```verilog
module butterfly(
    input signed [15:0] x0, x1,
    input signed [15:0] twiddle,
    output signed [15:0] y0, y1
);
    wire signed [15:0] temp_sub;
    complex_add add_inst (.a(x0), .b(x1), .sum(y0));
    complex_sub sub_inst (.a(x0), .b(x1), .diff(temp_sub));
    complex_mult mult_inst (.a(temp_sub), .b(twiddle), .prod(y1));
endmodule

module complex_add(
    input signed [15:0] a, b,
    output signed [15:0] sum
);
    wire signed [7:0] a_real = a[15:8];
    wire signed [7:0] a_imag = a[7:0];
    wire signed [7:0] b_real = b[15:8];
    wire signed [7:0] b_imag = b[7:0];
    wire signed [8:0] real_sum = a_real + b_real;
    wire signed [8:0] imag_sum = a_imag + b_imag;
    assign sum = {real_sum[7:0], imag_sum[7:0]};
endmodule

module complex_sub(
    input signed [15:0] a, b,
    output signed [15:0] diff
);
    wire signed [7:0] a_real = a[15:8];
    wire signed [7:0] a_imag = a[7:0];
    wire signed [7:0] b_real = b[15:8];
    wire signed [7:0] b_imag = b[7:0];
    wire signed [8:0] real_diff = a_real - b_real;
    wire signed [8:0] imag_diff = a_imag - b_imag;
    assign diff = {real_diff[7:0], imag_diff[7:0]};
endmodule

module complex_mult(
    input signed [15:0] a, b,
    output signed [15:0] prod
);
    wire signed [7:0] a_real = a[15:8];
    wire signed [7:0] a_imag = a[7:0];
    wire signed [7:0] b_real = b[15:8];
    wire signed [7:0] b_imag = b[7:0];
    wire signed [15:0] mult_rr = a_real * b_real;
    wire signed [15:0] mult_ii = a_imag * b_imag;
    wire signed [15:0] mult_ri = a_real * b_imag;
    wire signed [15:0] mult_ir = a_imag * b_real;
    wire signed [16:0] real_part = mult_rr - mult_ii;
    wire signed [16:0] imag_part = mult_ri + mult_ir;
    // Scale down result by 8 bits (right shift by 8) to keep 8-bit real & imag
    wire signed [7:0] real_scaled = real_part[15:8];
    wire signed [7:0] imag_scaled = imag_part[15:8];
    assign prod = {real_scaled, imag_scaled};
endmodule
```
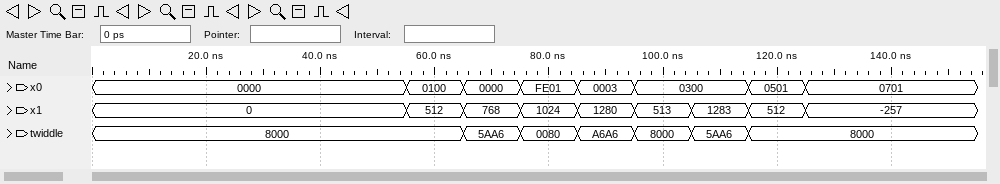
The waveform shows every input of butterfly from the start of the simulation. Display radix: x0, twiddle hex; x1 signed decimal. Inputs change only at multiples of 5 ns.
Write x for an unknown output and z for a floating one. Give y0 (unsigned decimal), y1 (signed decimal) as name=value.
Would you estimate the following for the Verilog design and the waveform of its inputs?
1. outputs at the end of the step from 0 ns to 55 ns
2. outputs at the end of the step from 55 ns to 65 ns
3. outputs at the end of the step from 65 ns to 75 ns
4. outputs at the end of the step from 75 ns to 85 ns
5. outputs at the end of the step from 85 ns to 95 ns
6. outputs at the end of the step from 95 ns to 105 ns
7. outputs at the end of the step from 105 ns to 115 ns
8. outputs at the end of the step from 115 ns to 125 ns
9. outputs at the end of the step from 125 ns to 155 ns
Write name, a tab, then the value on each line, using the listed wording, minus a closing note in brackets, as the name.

outputs at the end of the step from 0 ns to 55 ns	y0=0, y1=0
outputs at the end of the step from 55 ns to 65 ns	y0=768, y1=0
outputs at the end of the step from 65 ns to 75 ns	y0=768, y1=-511
outputs at the end of the step from 75 ns to 85 ns	y0=513, y1=3
outputs at the end of the step from 85 ns to 95 ns	y0=1283, y1=512
outputs at the end of the step from 95 ns to 105 ns	y0=1281, y1=-256
outputs at the end of the step from 105 ns to 115 ns	y0=2051, y1=-257
outputs at the end of the step from 115 ns to 125 ns	y0=1793, y1=-257
outputs at the end of the step from 125 ns to 155 ns	y0=1280, y1=-1025
